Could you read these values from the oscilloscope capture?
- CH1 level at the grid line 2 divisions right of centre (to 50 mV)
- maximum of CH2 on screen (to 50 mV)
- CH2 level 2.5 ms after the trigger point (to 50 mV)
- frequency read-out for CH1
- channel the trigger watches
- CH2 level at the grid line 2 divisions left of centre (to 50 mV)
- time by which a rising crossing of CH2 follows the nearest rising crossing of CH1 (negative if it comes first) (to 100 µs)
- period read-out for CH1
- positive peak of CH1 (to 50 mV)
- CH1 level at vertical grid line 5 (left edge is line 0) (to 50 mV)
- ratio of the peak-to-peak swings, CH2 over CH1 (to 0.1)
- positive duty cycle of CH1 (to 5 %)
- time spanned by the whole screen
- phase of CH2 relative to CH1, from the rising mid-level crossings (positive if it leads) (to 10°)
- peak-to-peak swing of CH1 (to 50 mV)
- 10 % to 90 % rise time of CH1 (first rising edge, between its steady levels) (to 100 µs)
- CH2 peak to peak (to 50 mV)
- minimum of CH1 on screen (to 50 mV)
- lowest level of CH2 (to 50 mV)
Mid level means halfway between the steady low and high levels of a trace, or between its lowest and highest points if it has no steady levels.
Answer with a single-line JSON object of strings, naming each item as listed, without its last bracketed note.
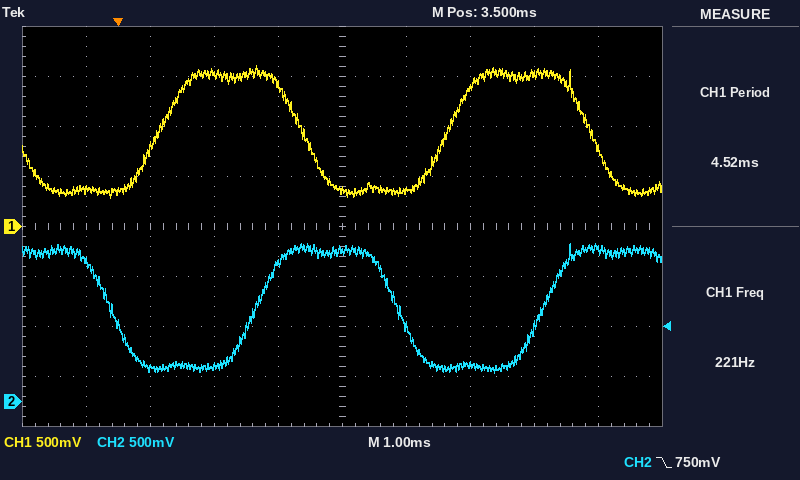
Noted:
{"CH1 level at the grid line 2 divisions right of centre": "1.40 V", "maximum of CH2 on screen": "1.60 V", "CH2 level 2.5 ms after the trigger point": "1.40 V", "frequency read-out for CH1": "221 Hz", "channel the trigger watches": "CH2", "CH2 level at the grid line 2 divisions left of centre": "350 mV", "time by which a rising crossing of CH2 follows the nearest rising crossing of CH1 (negative if it comes first)": "+1.5 ms", "period read-out for CH1": "4.52 ms", "positive peak of CH1": "1.60 V", "CH1 level at vertical grid line 5 (left edge is line 0)": "350 mV", "ratio of the peak-to-peak swings, CH2 over CH1": "1.0", "positive duty cycle of CH1": "50 %", "time spanned by the whole screen": "10 ms", "phase of CH2 relative to CH1, from the rising mid-level crossings (positive if it leads)": "-120°", "peak-to-peak swing of CH1": "1.30 V", "10 % to 90 % rise time of CH1 (first rising edge, between its steady levels)": "800 µs", "CH2 peak to peak": "1.30 V", "minimum of CH1 on screen": "300 mV", "lowest level of CH2": "300 mV"}
